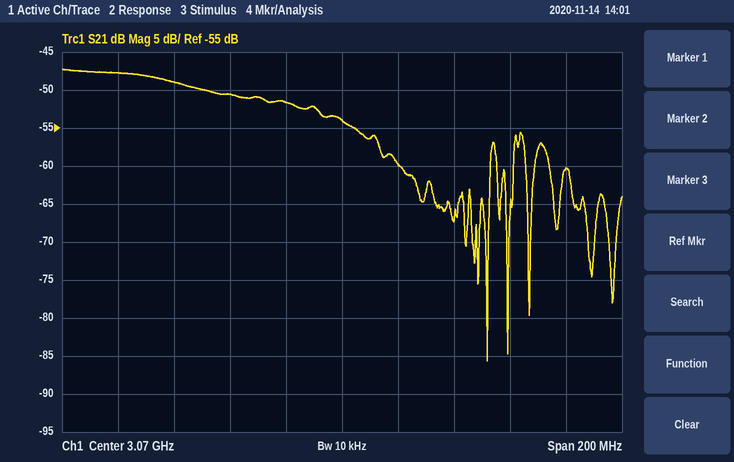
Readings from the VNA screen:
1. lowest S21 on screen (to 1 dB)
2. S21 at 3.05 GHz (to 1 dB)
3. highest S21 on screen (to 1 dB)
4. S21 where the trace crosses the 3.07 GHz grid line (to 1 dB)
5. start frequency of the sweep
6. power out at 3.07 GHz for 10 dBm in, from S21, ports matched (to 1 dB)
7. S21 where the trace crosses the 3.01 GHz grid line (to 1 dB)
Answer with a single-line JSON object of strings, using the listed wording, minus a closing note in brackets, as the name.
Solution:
{"lowest S21 on screen": "-86 dB", "S21 at 3.05 GHz": "-52 dB", "highest S21 on screen": "-47 dB", "S21 where the trace crosses the 3.07 GHz grid line": "-54 dB", "start frequency of the sweep": "2.97 GHz", "power out at 3.07 GHz for 10 dBm in, from S21, ports matched": "-44 dBm", "S21 where the trace crosses the 3.01 GHz grid line": "-49 dB"}
